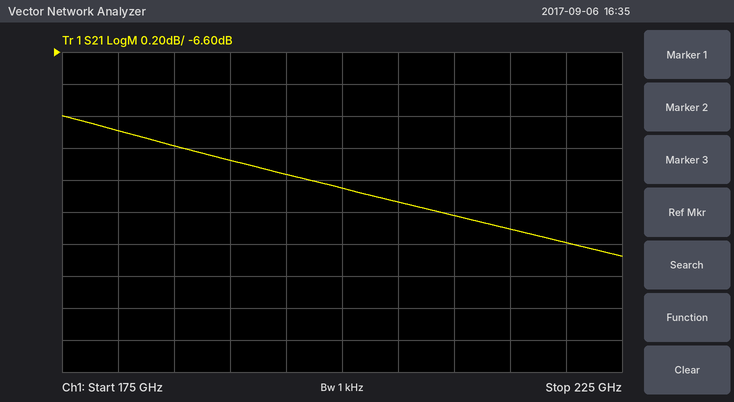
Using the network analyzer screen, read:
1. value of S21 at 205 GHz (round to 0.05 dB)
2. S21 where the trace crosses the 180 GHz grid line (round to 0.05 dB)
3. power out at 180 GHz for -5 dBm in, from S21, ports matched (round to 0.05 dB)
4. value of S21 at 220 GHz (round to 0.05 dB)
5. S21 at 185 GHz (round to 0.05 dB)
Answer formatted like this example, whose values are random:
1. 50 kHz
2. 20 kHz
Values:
1. -7.55 dB
2. -7.10 dB
3. -12.10 dBm
4. -7.80 dB
5. -7.20 dB
